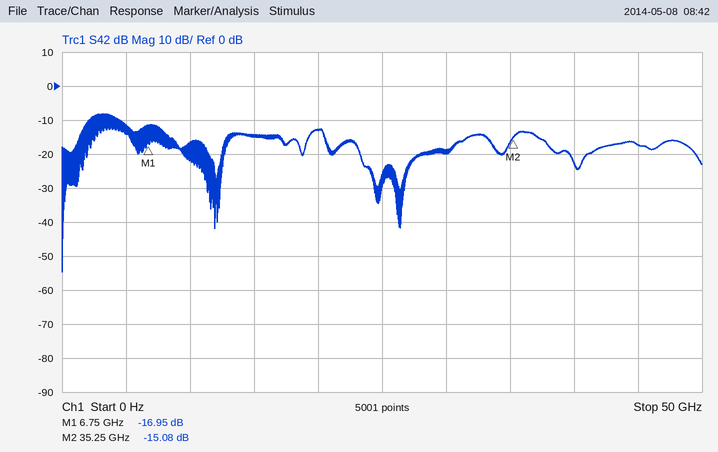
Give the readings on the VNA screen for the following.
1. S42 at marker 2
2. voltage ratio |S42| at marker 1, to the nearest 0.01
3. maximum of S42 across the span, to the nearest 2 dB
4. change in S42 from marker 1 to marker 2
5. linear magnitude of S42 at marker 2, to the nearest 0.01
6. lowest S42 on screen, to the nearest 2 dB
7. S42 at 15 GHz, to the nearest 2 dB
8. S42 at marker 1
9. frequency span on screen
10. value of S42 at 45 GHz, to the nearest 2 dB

-15.08 dB
0.14
-8 dB
1.87 dB
0.18
-54 dB
-14 dB
-16.95 dB
50 GHz
-18 dB
